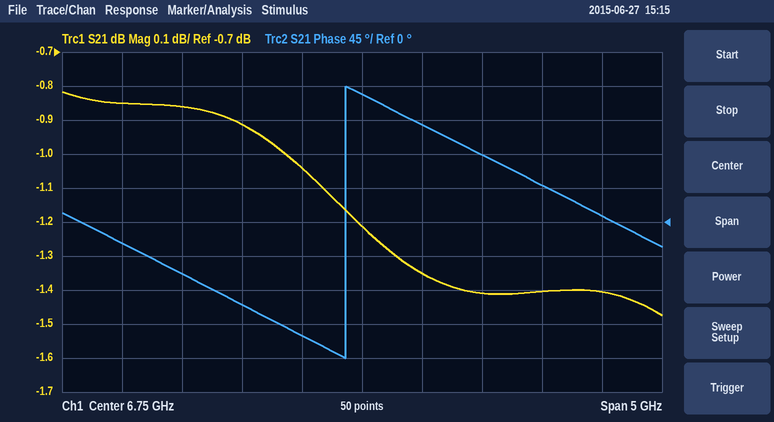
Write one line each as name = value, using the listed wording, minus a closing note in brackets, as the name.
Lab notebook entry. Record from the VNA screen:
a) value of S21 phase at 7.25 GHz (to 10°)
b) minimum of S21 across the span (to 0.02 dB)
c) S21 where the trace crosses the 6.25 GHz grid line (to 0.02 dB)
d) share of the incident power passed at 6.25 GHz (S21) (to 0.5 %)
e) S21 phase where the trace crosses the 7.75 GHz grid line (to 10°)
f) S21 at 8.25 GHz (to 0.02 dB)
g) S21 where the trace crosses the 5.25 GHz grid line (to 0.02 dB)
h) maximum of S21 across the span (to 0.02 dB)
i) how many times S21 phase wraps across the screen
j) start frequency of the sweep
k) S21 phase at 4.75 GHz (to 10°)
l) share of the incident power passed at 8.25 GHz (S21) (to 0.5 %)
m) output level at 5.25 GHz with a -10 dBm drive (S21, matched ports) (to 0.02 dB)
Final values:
value of S21 phase at 7.25 GHz = 130°
minimum of S21 across the span = -1.48 dB
S21 where the trace crosses the 6.25 GHz grid line = -1.04 dB
share of the incident power passed at 6.25 GHz (S21) = 78.5 %
S21 phase where the trace crosses the 7.75 GHz grid line = 90°
S21 at 8.25 GHz = -1.40 dB
S21 where the trace crosses the 5.25 GHz grid line = -0.86 dB
maximum of S21 across the span = -0.82 dB
how many times S21 phase wraps across the screen = 1
start frequency of the sweep = 4.25 GHz
S21 phase at 4.75 GHz = -30°
share of the incident power passed at 8.25 GHz (S21) = 72.5 %
output level at 5.25 GHz with a -10 dBm drive (S21, matched ports) = -10.86 dBm
